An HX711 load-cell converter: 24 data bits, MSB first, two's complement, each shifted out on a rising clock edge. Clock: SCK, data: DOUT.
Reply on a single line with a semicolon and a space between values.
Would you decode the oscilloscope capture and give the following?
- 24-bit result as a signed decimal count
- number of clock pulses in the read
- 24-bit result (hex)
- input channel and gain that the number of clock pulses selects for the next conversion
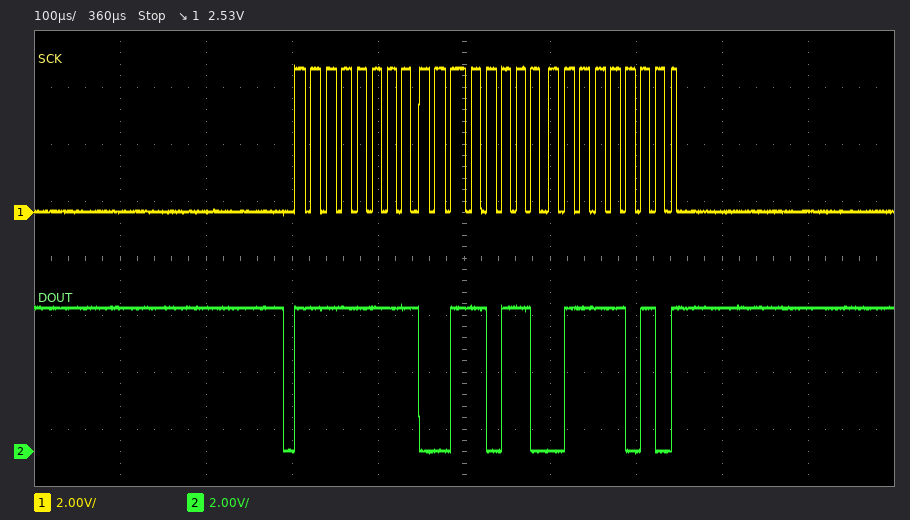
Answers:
-51590; 25; 0xFF367A; channel A, gain 128
